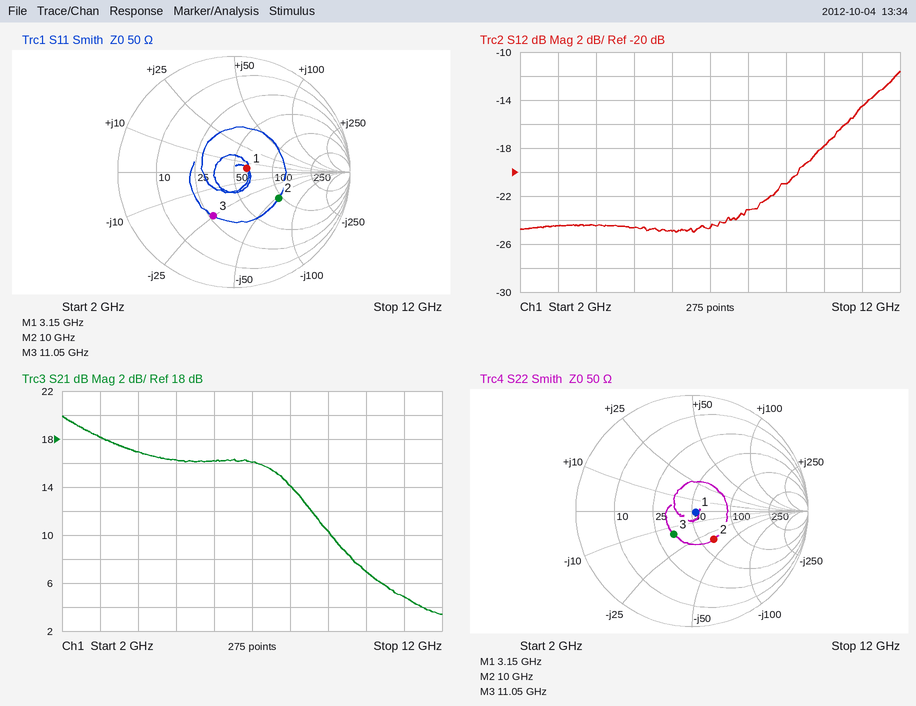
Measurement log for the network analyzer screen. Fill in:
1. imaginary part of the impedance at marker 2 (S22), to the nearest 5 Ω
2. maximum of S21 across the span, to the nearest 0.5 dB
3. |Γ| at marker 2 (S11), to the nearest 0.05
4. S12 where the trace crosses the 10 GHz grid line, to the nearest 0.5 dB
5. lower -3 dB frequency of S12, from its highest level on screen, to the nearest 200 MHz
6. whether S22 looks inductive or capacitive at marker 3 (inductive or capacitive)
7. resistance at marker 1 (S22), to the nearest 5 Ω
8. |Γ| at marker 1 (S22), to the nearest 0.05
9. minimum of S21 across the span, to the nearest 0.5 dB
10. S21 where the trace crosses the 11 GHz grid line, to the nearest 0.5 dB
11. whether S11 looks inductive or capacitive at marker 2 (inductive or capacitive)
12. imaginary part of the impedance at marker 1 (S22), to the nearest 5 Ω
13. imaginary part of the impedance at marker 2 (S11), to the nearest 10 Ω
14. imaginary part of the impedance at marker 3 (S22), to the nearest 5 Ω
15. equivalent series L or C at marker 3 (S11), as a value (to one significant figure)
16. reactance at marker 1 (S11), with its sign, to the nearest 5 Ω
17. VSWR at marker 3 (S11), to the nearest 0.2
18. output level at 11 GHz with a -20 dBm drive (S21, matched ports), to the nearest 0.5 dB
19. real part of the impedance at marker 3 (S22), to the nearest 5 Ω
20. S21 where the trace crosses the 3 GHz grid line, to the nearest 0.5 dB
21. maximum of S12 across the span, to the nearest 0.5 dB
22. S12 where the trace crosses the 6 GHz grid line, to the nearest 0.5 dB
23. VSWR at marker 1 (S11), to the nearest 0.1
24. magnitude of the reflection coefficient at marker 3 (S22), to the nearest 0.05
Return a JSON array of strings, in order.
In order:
["-35 Ω", "20.0 dB", "0.45", "-18.0 dB", "11.0 GHz", "capacitive", "55 Ω", "0.05", "3.5 dB", "5.0 dB", "capacitive", "0 Ω", "-50 Ω", "-15 Ω", "600 fF", "+5 Ω", "2.4", "-15.0 dBm", "35 Ω", "18.0 dB", "-11.5 dB", "-25.0 dB", "1.3", "0.25"]
